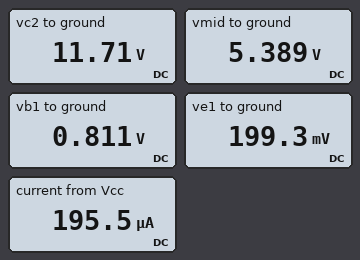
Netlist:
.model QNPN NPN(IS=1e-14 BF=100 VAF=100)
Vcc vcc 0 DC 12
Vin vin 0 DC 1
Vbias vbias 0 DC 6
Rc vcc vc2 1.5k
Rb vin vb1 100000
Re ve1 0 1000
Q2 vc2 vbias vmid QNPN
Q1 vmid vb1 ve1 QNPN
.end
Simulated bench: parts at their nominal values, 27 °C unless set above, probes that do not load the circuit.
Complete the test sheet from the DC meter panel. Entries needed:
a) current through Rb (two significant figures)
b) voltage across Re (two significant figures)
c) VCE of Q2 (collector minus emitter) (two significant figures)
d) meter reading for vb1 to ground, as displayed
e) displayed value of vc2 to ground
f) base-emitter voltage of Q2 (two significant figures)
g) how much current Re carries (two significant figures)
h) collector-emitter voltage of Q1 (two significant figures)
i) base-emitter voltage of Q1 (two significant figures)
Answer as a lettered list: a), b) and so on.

a) 1.9 µA
b) 200 mV
c) 6.3 V
d) 0.811 V
e) 11.71 V
f) 610 mV
g) 200 µA
h) 5.2 V
i) 610 mV
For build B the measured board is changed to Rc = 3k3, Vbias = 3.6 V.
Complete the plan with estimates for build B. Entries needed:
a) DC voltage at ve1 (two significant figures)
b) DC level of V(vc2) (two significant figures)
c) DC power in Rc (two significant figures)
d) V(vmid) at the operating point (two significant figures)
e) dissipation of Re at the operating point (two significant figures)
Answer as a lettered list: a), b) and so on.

a) 200 mV
b) 11 V
c) 120 µW
d) 3.0 V
e) 39 µW
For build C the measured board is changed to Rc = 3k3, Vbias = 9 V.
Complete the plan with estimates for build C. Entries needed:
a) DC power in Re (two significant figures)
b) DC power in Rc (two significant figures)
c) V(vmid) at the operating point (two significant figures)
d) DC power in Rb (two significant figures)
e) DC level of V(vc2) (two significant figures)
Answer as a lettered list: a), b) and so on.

a) 41 µW
b) 130 µW
c) 8.4 V
d) 350 nW
e) 11 V
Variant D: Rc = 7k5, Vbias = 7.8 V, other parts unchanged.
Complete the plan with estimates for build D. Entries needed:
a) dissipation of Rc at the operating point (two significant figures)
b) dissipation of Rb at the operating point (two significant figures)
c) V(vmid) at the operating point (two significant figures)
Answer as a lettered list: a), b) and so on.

a) 290 µW
b) 350 nW
c) 7.2 V
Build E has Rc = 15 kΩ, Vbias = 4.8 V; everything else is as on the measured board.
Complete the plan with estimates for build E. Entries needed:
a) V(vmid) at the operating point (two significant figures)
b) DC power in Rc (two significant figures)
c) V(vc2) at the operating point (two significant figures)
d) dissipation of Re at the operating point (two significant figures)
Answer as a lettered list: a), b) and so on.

a) 4.2 V
b) 570 µW
c) 9.1 V
d) 39 µW
